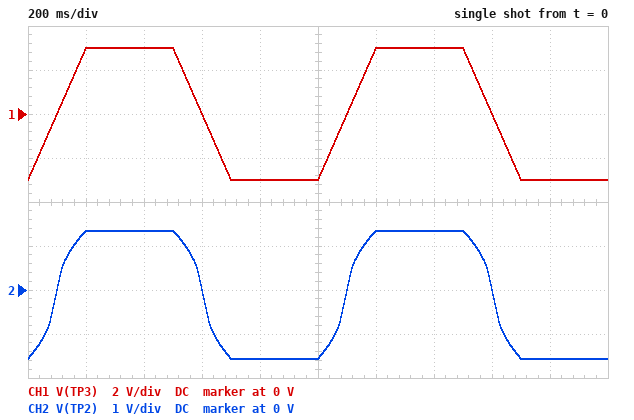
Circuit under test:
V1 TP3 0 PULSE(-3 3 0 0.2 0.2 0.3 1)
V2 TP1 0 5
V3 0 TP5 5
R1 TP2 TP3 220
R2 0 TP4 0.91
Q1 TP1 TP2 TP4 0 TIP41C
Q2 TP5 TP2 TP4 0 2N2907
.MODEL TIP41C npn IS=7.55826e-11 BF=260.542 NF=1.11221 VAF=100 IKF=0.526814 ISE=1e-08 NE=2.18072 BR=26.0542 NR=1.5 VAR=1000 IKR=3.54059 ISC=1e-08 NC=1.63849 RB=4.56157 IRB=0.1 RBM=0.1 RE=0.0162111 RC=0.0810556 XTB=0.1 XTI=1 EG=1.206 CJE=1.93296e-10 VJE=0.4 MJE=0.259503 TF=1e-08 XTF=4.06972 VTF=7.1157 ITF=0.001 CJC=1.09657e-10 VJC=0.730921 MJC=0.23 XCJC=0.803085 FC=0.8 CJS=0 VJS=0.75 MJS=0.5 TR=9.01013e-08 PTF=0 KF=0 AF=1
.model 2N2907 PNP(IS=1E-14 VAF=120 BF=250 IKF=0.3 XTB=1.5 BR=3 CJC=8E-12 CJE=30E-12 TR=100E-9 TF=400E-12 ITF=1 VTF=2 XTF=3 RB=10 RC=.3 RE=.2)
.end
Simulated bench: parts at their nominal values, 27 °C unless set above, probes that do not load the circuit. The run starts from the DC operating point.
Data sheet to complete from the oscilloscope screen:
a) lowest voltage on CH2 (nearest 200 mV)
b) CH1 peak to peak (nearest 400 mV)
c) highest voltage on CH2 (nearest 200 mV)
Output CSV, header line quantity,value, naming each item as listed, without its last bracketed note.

quantity,value
lowest voltage on CH2,-1.6 V
CH1 peak to peak,6.0 V
highest voltage on CH2,1.4 V
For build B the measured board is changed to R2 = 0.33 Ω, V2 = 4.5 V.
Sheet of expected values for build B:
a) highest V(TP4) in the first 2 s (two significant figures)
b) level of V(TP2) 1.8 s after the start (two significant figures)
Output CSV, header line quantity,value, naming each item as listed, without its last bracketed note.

quantity,value
highest V(TP4) in the first 2 s,260 mV
level of V(TP2) 1.8 s after the start,-1.3 V
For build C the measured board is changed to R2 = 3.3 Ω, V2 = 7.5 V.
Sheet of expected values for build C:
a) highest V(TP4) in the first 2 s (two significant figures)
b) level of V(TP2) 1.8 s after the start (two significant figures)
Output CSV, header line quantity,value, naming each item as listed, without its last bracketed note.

quantity,value
highest V(TP4) in the first 2 s,1.4 V
level of V(TP2) 1.8 s after the start,-2.2 V
